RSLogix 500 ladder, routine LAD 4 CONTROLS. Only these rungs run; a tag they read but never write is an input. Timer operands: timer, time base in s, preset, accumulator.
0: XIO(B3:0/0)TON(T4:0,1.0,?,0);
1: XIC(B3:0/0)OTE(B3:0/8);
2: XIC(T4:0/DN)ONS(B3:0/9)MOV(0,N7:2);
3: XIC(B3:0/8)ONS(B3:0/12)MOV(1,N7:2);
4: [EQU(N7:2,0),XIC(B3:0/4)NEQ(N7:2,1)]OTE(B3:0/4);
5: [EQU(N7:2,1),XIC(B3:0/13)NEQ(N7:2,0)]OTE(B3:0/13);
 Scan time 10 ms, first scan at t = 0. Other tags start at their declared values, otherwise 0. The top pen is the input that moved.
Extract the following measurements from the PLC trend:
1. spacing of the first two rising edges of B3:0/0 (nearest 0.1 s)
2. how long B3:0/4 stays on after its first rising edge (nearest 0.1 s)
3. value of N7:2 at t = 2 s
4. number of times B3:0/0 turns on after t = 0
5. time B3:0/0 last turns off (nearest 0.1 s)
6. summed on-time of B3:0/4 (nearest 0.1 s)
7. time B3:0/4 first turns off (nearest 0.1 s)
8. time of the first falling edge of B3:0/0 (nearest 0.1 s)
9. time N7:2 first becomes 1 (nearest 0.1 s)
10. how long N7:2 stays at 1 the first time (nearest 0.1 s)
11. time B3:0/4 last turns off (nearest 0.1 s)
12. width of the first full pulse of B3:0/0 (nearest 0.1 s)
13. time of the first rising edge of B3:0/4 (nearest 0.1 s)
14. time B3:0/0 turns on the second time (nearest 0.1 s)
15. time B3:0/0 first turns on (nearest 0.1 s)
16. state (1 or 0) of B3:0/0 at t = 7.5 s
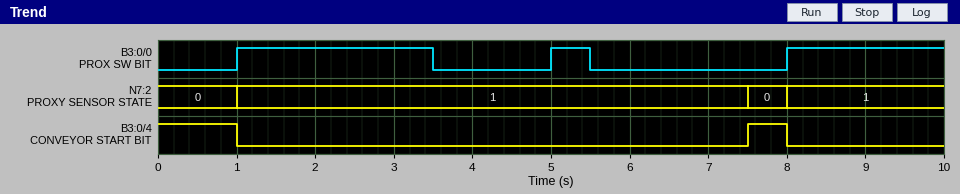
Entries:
4.0 s
0.5 s
1
3
5.5 s
1.5 s
1.0 s
3.5 s
1.0 s
6.5 s
8.0 s
2.5 s
7.5 s
5.0 s
1.0 s
0
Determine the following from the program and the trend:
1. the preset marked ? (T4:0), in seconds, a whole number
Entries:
2 s
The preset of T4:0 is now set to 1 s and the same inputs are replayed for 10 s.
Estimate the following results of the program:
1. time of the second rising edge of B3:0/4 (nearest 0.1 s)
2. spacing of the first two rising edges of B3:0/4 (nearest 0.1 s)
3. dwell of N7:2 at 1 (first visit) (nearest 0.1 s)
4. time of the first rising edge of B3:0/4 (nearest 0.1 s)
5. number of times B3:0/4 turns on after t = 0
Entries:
6.5 s
2.0 s
3.5 s
4.5 s
2
